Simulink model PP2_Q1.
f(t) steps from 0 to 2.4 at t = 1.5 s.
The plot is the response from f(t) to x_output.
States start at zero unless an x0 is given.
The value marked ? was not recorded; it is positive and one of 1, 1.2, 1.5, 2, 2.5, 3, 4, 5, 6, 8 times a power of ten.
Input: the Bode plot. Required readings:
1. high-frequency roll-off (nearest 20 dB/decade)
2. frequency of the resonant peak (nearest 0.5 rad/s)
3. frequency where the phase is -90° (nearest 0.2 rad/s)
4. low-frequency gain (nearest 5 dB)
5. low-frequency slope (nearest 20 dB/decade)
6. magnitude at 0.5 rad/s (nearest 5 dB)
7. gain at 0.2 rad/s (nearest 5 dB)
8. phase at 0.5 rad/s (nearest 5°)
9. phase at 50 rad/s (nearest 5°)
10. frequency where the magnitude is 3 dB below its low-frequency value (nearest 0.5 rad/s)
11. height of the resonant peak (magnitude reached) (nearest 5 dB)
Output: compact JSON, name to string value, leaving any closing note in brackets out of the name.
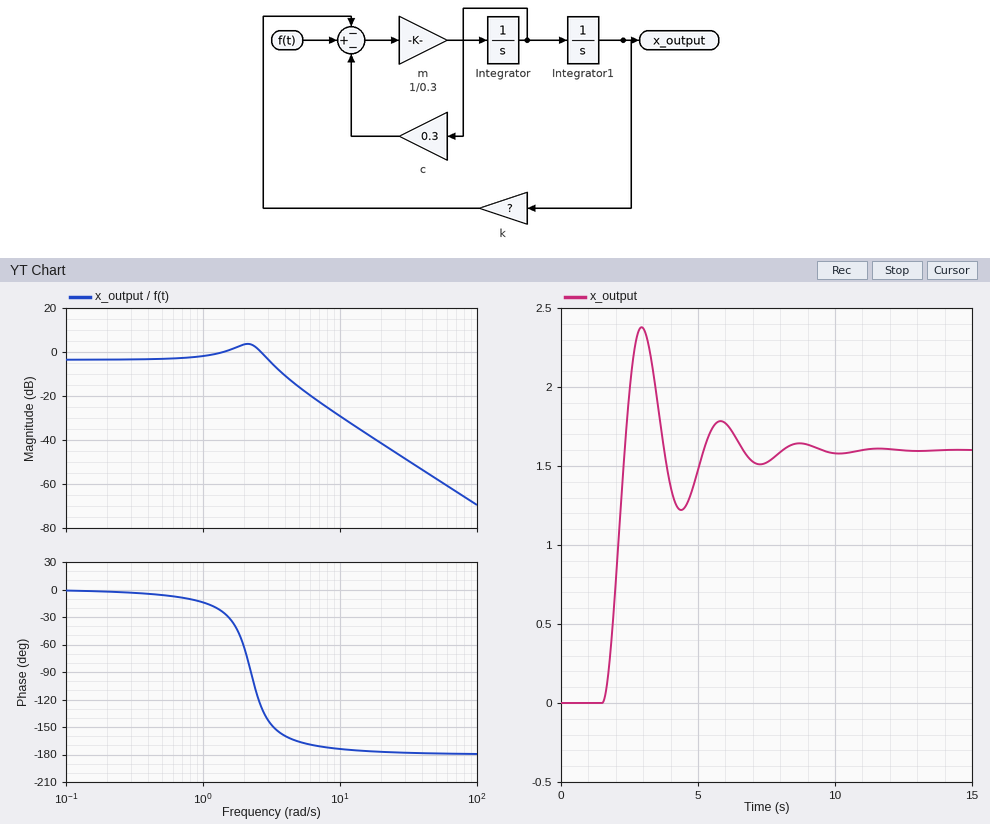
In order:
{"high-frequency roll-off": "-40 dB/decade", "frequency of the resonant peak": "2.0 rad/s", "frequency where the phase is -90°": "2.2 rad/s", "low-frequency gain": "-5 dB", "low-frequency slope": "0 dB/decade", "magnitude at 0.5 rad/s": "-5 dB", "gain at 0.2 rad/s": "-5 dB", "phase at 0.5 rad/s": "-5°", "phase at 50 rad/s": "-180°", "frequency where the magnitude is 3 dB below its low-frequency value": "3.5 rad/s", "height of the resonant peak (magnitude reached)": "5 dB"}
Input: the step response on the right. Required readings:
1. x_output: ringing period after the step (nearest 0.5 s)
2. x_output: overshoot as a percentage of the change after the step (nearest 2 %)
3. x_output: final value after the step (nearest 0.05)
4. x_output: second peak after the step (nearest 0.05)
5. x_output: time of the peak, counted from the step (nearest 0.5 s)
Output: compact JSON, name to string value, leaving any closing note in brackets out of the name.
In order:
{"x_output: ringing period after the step": "3.0 s", "x_output: overshoot as a percentage of the change after the step": "48 %", "x_output: final value after the step": "1.60", "x_output: second peak after the step": "1.80", "x_output: time of the peak, counted from the step": "1.5 s"}
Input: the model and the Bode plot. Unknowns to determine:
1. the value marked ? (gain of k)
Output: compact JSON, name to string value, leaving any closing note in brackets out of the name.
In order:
{"the value marked ?": "1.5"}
